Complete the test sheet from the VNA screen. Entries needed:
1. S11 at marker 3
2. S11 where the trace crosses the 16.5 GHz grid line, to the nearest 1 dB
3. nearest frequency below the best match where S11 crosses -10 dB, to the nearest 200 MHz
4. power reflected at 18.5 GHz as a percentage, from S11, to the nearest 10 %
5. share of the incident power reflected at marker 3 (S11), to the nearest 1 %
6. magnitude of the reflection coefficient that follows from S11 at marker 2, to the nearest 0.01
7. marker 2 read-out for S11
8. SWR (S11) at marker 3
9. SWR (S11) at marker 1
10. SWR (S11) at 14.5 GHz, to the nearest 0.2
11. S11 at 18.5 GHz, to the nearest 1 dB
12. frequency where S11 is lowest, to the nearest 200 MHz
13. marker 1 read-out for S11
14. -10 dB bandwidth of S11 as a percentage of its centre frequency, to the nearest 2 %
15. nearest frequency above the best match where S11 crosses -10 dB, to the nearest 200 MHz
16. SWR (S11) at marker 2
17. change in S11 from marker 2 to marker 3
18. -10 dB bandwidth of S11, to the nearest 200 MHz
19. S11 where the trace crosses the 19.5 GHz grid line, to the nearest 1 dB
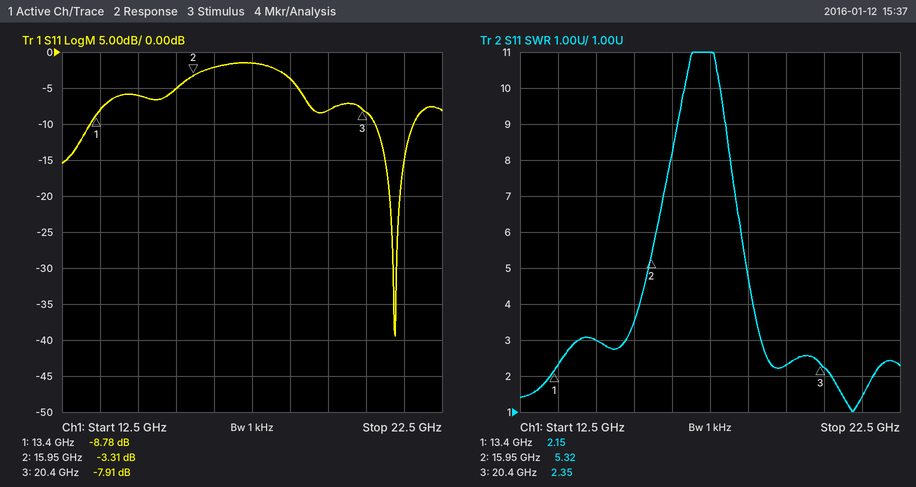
-7.91 dB
-2 dB
20.8 GHz
40 %
16 %
0.68
-3.31 dB
2.35
2.15
3.0
-4 dB
21.2 GHz
-8.78 dB
4 %
21.8 GHz
5.32
-4.60 dB
1.0 GHz
-8 dB
